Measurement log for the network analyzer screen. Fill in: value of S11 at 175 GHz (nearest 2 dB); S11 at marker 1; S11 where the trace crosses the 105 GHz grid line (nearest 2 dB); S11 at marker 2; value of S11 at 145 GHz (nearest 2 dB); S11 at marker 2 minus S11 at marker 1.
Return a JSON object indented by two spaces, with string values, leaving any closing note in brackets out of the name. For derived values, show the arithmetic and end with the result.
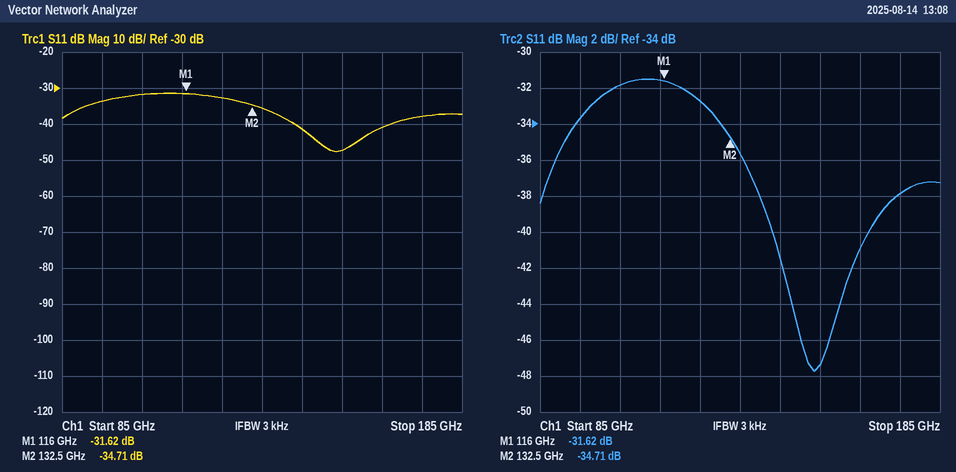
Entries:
{
  "value of S11 at 175 GHz": "-38 dB",
  "S11 at marker 1": "-31.62 dB",
  "S11 where the trace crosses the 105 GHz grid line": "-32 dB",
  "S11 at marker 2": "-34.71 dB",
  "value of S11 at 145 GHz": "-42 dB",
  "S11 at marker 2 minus S11 at marker 1": "-34.71 − (-31.62) = -3.09 dB"
}
